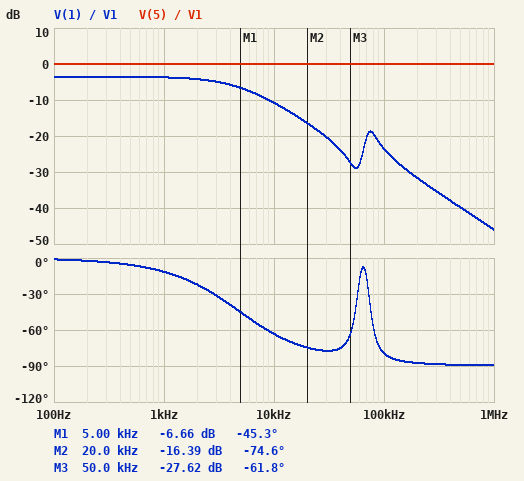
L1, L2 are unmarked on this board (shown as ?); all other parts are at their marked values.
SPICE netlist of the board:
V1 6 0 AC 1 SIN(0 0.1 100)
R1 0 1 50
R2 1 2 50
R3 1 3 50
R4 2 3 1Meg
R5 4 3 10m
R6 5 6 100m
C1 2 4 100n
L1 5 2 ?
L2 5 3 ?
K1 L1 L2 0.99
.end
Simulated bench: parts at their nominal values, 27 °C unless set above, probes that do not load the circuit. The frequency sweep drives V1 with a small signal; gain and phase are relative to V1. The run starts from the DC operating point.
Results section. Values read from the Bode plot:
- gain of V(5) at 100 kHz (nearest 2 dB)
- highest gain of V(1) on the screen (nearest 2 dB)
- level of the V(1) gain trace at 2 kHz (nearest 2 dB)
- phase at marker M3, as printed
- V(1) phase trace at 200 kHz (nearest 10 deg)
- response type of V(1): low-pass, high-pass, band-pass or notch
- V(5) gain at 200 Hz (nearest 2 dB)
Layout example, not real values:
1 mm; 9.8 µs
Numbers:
0 dB; -4 dB; -4 dB; -61.8 deg; -90 deg; low-pass; 0 dB
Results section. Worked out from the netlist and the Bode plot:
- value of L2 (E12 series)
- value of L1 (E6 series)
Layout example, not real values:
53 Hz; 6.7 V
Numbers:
2.7 mH; 2.2 mH
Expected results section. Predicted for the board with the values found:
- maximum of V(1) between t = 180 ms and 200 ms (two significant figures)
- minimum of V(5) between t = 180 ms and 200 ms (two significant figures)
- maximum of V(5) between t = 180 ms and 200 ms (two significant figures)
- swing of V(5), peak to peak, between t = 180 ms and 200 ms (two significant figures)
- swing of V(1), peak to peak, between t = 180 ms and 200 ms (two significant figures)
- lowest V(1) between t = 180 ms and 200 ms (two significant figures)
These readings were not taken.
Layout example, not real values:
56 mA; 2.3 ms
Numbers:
67 mV; -100 mV; 100 mV; 200 mV; 130 mV; -67 mV
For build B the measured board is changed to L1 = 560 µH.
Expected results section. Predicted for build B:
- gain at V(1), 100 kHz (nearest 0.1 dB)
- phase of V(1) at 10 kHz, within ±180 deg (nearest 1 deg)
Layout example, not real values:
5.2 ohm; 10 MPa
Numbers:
-4.0 dB; -31 deg
